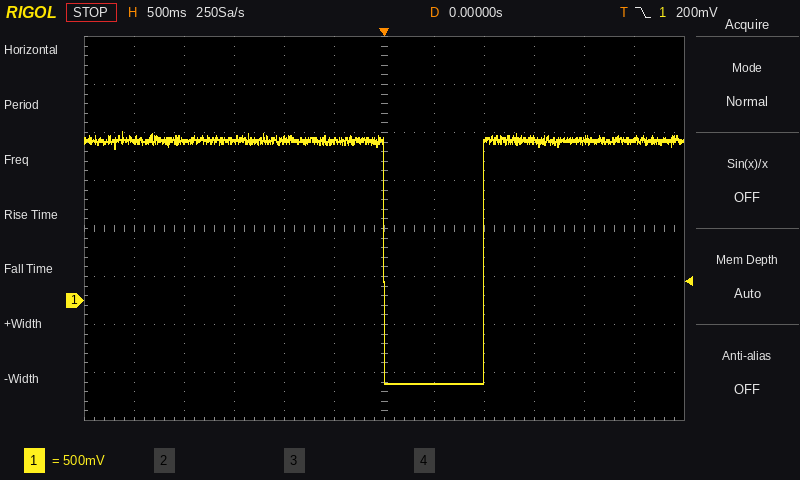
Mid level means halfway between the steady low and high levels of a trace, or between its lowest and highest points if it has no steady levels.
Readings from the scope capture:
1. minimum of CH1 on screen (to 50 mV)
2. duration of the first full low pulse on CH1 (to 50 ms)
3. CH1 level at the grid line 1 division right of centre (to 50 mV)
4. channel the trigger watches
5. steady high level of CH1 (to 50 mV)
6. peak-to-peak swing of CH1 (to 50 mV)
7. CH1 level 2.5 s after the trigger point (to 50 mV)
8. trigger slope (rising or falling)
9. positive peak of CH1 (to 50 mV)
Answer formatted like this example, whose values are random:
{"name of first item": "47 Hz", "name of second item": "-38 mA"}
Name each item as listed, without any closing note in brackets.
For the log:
{"minimum of CH1 on screen": "-850 mV", "duration of the first full low pulse on CH1": "1.00 s", "CH1 level at the grid line 1 division right of centre": "-850 mV", "channel the trigger watches": "CH1", "steady high level of CH1": "1.65 V", "peak-to-peak swing of CH1": "2.60 V", "CH1 level 2.5 s after the trigger point": "1.70 V", "trigger slope": "falling", "positive peak of CH1": "1.75 V"}
